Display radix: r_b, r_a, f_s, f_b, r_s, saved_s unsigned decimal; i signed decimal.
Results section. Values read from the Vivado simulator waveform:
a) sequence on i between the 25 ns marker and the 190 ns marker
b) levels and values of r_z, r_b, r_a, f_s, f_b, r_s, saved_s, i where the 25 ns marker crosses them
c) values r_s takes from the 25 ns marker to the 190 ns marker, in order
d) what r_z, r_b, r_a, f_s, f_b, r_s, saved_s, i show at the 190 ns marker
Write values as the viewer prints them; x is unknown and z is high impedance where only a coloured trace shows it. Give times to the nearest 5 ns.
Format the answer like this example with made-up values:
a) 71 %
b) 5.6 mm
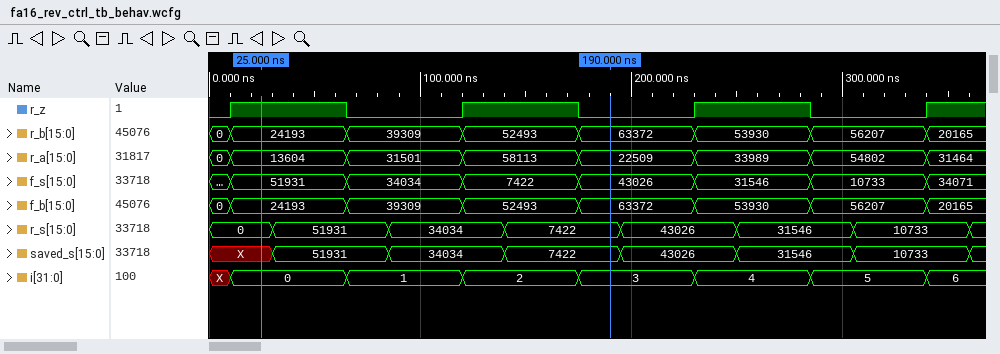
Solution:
a) 0, 1, 2, 3
b) r_z=1, r_b=24193, r_a=13604, f_s=51931, f_b=24193, r_s=0, saved_s=X, i=0
c) 0, 51931, 34034, 7422
d) r_z=0, r_b=63372, r_a=22509, f_s=43026, f_b=63372, r_s=7422, saved_s=7422, i=3
